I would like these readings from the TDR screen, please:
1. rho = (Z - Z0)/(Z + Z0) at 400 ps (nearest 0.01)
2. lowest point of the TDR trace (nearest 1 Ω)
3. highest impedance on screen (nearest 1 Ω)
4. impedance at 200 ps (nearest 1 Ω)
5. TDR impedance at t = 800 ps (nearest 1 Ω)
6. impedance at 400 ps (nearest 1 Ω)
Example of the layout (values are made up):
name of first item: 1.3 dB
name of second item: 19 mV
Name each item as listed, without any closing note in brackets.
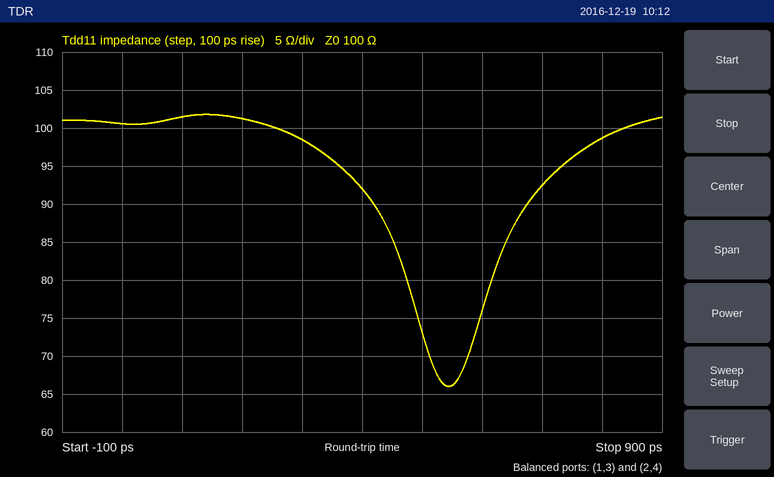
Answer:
rho = (Z - Z0)/(Z + Z0) at 400 ps: -0.04
lowest point of the TDR trace: 66 Ω
highest impedance on screen: 102 Ω
impedance at 200 ps: 101 Ω
TDR impedance at t = 800 ps: 99 Ω
impedance at 400 ps: 92 Ω
